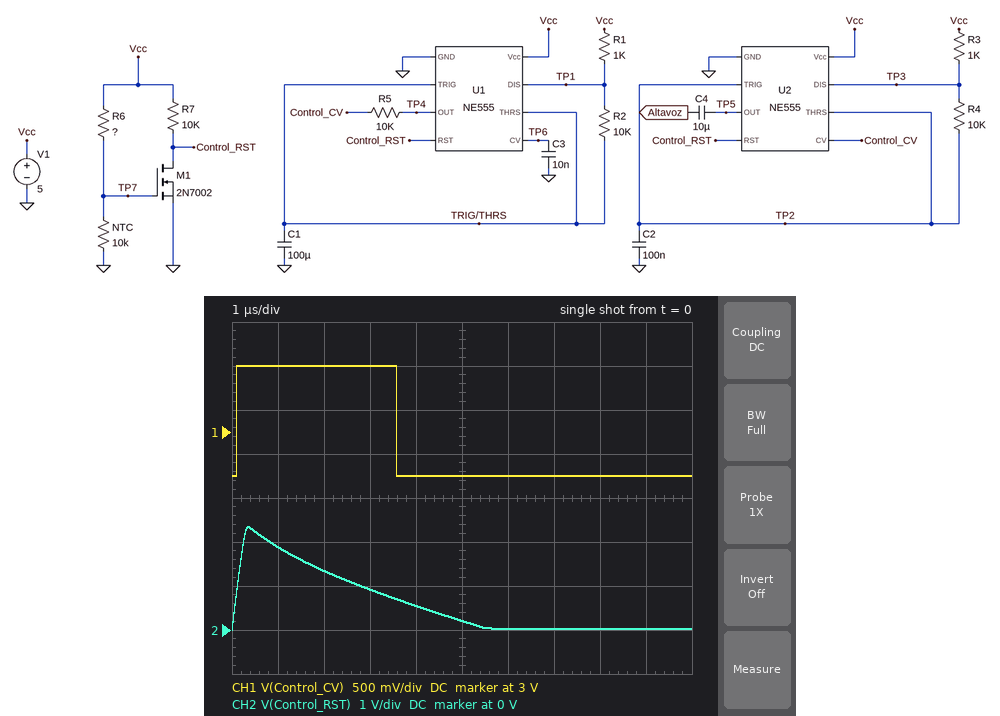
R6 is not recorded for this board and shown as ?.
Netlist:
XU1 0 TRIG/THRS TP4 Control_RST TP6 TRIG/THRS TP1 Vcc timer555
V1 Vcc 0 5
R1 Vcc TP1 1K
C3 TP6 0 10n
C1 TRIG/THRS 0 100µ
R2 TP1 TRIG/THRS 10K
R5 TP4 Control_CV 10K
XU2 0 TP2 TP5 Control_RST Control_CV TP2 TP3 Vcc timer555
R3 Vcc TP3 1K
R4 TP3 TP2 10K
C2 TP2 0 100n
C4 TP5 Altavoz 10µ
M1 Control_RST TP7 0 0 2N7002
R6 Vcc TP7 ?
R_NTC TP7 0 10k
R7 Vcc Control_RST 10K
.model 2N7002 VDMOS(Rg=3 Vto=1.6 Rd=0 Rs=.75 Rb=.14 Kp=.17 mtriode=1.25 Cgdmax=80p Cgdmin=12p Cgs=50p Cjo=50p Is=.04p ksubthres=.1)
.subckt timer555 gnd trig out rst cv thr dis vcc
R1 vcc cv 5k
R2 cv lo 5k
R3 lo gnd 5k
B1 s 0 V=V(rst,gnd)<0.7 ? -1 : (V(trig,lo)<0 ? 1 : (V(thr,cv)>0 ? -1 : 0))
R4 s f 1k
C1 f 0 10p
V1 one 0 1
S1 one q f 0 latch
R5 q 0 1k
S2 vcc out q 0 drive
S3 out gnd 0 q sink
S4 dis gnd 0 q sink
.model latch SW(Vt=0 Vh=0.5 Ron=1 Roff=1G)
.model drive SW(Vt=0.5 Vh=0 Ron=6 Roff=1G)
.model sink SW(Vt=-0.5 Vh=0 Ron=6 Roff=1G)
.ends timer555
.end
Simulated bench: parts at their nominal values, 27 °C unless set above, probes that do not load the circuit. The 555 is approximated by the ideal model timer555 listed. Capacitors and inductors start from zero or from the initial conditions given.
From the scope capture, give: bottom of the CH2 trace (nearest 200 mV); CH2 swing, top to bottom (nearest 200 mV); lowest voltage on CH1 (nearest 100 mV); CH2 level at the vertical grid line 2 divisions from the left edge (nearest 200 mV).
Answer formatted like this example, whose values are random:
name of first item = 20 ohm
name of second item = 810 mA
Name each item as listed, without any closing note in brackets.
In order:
bottom of the CH2 trace = 0 V
CH2 swing, top to bottom = 2.4 V
lowest voltage on CH1 = 2.5 V
CH2 level at the vertical grid line 2 divisions from the left edge = 1.4 V
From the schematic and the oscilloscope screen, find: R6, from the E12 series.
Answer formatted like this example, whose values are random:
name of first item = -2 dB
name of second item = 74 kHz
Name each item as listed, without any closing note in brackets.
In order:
R6, from the E12 series = 18 kΩ
